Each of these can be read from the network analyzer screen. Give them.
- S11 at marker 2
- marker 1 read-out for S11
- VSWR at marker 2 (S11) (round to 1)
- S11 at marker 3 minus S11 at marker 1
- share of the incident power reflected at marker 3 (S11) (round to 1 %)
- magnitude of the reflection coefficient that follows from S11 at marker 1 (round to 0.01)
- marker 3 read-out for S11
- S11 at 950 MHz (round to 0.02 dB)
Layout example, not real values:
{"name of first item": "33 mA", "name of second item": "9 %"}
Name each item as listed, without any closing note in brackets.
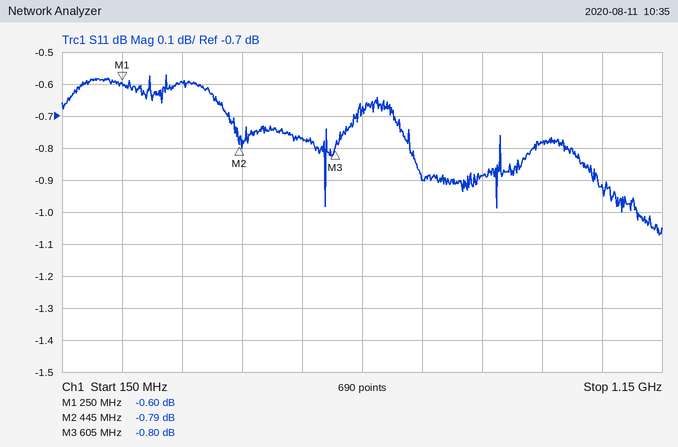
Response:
{"S11 at marker 2": "-0.79 dB", "marker 1 read-out for S11": "-0.60 dB", "VSWR at marker 2 (S11)": "22", "S11 at marker 3 minus S11 at marker 1": "-0.20 dB", "share of the incident power reflected at marker 3 (S11)": "83 %", "magnitude of the reflection coefficient that follows from S11 at marker 1": "0.93", "marker 3 read-out for S11": "-0.80 dB", "S11 at 950 MHz": "-0.78 dB"}
